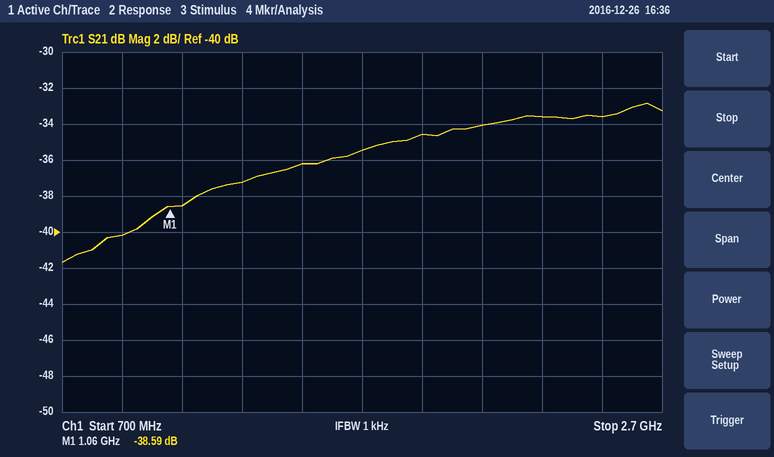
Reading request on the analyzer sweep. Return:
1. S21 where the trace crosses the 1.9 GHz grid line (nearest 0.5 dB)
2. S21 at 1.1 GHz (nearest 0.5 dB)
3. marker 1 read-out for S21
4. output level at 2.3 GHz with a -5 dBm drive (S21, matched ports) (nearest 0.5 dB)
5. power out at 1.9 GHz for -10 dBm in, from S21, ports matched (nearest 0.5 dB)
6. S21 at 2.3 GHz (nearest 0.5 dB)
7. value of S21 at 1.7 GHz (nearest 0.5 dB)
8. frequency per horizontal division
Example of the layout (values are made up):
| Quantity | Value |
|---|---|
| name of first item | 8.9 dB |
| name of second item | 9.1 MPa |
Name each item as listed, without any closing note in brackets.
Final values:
| Quantity | Value |
|---|---|
| S21 where the trace crosses the 1.9 GHz grid line | -34.5 dB |
| S21 at 1.1 GHz | -38.5 dB |
| marker 1 read-out for S21 | -38.59 dB |
| output level at 2.3 GHz with a -5 dBm drive (S21, matched ports) | -38.5 dBm |
| power out at 1.9 GHz for -10 dBm in, from S21, ports matched | -44.5 dBm |
| S21 at 2.3 GHz | -33.5 dB |
| value of S21 at 1.7 GHz | -35.5 dB |
| frequency per horizontal division | 200 MHz |
